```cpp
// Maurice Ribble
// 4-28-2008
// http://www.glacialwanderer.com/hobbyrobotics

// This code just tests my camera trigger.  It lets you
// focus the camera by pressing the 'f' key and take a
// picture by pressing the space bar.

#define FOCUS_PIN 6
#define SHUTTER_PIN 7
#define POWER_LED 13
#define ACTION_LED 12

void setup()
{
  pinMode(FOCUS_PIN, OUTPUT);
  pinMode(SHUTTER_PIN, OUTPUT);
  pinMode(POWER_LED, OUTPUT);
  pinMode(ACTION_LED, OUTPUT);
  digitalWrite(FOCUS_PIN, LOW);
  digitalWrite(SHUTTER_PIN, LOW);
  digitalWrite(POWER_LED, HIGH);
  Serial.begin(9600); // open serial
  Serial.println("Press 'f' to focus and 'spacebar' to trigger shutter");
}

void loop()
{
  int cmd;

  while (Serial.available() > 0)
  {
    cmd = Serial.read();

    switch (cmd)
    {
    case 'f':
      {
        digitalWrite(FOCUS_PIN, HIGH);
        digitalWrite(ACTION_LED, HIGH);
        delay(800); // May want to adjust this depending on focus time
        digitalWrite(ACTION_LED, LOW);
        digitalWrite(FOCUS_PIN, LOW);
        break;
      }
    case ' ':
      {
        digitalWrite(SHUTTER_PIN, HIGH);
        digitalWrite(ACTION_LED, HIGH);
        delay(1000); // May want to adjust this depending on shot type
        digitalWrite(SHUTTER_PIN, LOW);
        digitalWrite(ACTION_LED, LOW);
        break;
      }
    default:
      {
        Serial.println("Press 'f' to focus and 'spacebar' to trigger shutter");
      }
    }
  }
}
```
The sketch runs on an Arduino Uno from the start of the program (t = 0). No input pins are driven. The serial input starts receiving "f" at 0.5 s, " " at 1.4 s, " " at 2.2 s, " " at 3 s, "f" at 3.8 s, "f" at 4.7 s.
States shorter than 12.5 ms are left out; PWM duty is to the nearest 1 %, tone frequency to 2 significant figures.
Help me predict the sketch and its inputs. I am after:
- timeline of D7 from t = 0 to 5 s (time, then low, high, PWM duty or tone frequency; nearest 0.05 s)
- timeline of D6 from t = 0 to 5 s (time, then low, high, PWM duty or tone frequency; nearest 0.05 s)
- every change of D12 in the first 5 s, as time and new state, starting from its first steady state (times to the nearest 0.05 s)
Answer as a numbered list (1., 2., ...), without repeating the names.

1. 0 s low; 1.4 s high; 4.4 s low
2. 0 s low; 0.5 s high; 1.3 s low; 4.4 s high
3. 0 s low; 0.5 s high; 1.3 s low; 1.4 s high
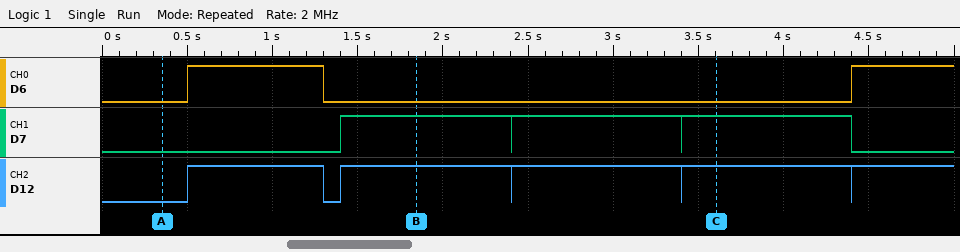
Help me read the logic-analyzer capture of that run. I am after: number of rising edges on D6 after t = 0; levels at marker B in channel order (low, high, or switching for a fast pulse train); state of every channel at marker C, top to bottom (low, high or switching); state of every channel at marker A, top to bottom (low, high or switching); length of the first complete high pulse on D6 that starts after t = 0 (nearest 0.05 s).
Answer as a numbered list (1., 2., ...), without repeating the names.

1. 2
2. D6 low, D7 high, D12 high
3. D6 low, D7 high, D12 high
4. D6 low, D7 low, D12 low
5. 0.80 s
